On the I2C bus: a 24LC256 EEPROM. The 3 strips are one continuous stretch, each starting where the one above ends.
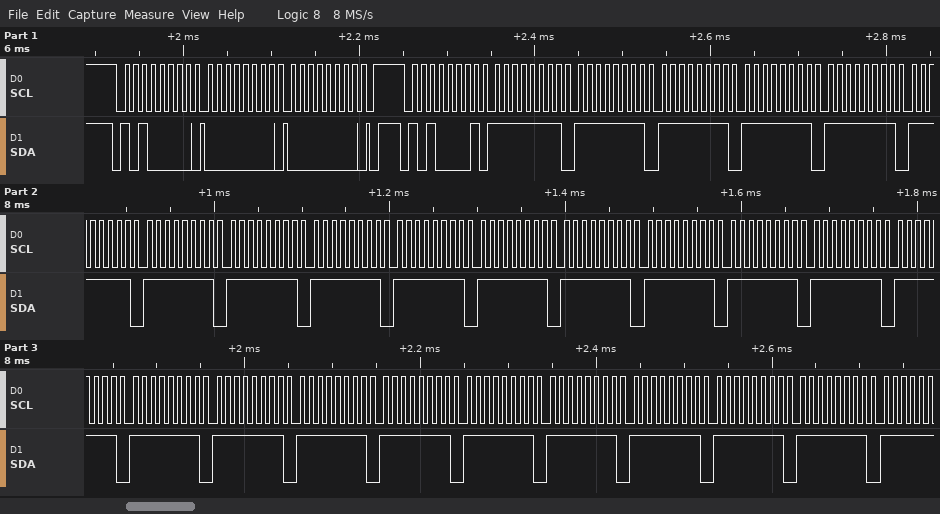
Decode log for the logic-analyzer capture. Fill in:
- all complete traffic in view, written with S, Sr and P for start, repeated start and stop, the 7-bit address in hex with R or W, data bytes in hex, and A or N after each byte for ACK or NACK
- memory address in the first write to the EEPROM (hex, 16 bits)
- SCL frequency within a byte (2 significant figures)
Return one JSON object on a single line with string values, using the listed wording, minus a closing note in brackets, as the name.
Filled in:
{"all complete traffic in view, written with S, Sr and P for start, repeated start and stop, the 7-bit address in hex with R or W, data bytes in hex, and A or N after each byte for ACK or NACK": "S 50W A 00 A 00 A P S 50R A FF A FF A FF A FF A FF A FF A FF A FF A FF A FF A FF A FF A FF A FF A FF A FF A FF A FF A FF A FF A FF A FF A FF A FF A FF A", "memory address in the first write to the EEPROM": "0x0000", "SCL frequency within a byte": "100 kHz"}
